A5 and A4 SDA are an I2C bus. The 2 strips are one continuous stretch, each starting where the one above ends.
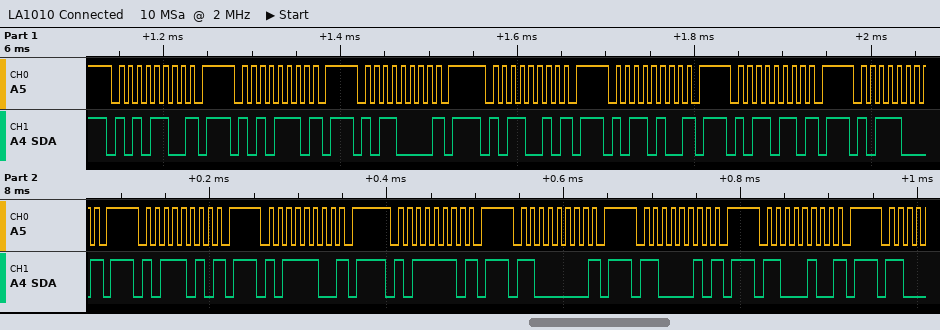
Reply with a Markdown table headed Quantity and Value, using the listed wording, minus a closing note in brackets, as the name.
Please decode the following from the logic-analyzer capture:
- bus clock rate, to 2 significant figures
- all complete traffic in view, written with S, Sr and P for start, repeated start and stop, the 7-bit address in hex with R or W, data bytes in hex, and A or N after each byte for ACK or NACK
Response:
| Quantity | Value |
|---|---|
| bus clock rate, to 2 significant figures | 100 kHz |
| all complete traffic in view, written with S, Sr and P for start, repeated start and stop, the 7-bit address in hex with R or W, data bytes in hex, and A or N after each byte for ACK or NACK | S 56W N P S 57W N P S 58W N P S 59W N P S 5AW N P S 5BW N P S 5CW N P S 5DW N P S 5EW N P S 5FW N P S 60W N P S 61W N P S 62W N P |
